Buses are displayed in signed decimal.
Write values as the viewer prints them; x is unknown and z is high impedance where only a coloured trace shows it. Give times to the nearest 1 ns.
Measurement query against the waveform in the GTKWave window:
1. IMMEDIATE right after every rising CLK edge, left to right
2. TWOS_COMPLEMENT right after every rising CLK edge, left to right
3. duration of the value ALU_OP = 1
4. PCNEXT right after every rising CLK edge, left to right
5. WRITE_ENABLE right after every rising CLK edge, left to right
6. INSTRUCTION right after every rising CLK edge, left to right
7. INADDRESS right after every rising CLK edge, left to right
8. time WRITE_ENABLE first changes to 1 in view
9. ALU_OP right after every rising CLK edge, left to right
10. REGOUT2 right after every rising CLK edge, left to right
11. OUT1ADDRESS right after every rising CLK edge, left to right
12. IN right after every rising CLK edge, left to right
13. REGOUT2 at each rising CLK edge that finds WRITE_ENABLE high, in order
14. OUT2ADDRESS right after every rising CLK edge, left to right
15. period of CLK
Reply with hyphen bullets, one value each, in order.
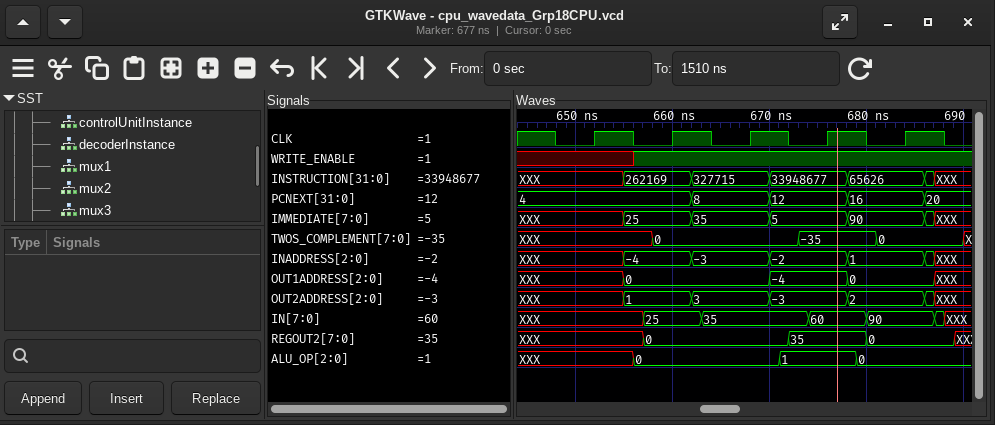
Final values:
- XXX, 25, 35, 5, 90
- XXX, 0, 0, -35, 0
- 8 ns
- 4, 4, 8, 12, 16
- x 1 1 1 1
- XXX, 262169, 327715, 33948677, 65626
- XXX, -4, -3, -2, 1
- 656 ns
- XXX, 0, 0, 1, 0
- XXX, 0, 0, 35, 0
- XXX, 0, 0, -4, 0
- XXX, 25, 35, 60, 90
- 0, 0, 35, 0
- XXX, 1, 3, -3, 2
- 8 ns
